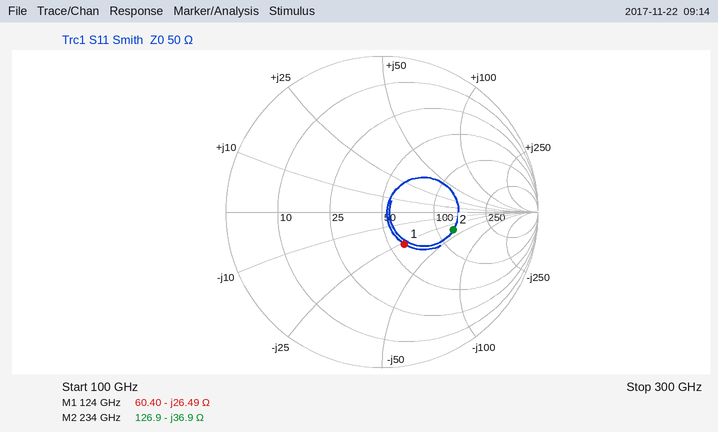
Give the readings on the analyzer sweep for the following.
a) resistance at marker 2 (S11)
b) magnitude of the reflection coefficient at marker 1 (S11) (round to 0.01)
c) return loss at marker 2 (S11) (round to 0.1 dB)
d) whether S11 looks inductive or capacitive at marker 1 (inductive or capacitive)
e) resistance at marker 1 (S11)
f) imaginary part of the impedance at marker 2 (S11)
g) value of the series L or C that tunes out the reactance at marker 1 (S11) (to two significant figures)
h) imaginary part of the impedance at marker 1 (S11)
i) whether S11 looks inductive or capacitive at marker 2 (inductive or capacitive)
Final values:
126.9 Ω
0.25
6.5 dB
capacitive
60.40 Ω
-36.9 Ω
34 pH
-26.49 Ω
capacitive
